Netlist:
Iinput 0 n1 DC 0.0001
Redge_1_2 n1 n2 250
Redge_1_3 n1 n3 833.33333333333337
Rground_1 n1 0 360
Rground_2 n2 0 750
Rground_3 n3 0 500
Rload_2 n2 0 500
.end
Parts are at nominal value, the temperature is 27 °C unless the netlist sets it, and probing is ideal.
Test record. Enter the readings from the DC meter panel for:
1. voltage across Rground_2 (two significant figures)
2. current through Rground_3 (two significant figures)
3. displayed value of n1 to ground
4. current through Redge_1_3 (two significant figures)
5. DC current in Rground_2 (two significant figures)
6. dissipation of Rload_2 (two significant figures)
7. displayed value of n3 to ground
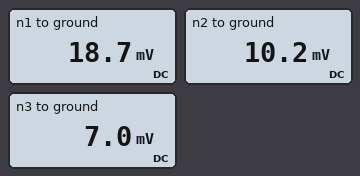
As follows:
10 mV
14 µA
18.7 mV
14 µA
14 µA
210 nW
7.0 mV
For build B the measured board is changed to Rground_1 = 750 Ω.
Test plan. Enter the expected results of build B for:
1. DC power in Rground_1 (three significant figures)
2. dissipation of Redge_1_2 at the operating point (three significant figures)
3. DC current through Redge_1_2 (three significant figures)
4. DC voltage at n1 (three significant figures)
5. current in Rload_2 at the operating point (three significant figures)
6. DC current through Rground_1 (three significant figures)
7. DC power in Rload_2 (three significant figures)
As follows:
876 nW
543 nW
46.6 µA
25.6 mV
28.0 µA
34.2 µA
391 nW
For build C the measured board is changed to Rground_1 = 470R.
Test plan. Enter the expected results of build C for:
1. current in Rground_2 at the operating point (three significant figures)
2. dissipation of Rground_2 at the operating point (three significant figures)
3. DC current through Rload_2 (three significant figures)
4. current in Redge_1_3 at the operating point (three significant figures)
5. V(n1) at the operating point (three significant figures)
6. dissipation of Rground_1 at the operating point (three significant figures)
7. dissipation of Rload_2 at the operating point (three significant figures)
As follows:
15.5 µA
180 nW
23.2 µA
16.0 µA
21.3 mV
965 nW
270 nW
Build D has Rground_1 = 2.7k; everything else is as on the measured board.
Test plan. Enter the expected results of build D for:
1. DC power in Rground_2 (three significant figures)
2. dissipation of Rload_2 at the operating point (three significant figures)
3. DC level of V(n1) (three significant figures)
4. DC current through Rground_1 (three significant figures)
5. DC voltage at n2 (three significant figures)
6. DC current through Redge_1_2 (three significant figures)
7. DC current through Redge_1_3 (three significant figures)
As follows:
459 nW
689 nW
34.0 mV
12.6 µA
18.6 mV
61.9 µA
25.5 µA
